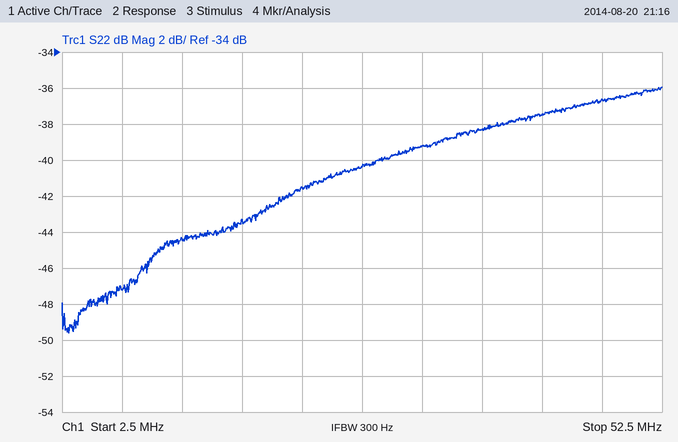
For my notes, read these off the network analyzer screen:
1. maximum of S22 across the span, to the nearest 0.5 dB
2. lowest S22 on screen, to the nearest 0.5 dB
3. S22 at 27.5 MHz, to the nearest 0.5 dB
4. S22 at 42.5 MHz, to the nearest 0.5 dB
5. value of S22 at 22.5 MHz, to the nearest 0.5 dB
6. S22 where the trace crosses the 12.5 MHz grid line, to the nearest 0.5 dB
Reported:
-36.0 dB
-49.5 dB
-40.5 dB
-37.5 dB
-41.5 dB
-44.5 dB
